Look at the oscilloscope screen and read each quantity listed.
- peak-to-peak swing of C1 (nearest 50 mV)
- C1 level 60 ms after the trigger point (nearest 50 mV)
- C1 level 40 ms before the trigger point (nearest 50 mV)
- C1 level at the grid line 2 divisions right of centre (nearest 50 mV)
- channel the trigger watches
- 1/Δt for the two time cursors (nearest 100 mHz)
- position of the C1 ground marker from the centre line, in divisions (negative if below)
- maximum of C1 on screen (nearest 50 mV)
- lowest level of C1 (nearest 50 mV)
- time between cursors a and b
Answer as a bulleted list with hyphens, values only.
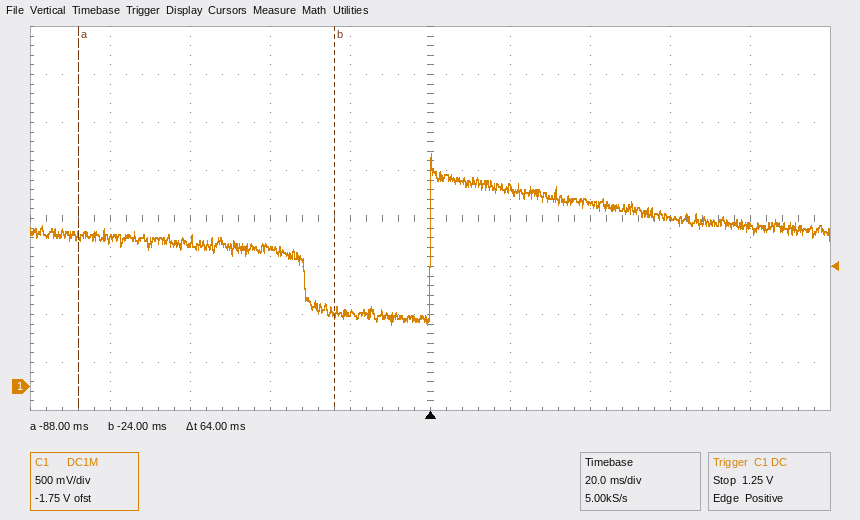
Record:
- 1.80 V
- 1.75 V
- 1.45 V
- 1.90 V
- C1
- 15.6 Hz
- -3.5 div
- 2.45 V
- 650 mV
- 64 ms
